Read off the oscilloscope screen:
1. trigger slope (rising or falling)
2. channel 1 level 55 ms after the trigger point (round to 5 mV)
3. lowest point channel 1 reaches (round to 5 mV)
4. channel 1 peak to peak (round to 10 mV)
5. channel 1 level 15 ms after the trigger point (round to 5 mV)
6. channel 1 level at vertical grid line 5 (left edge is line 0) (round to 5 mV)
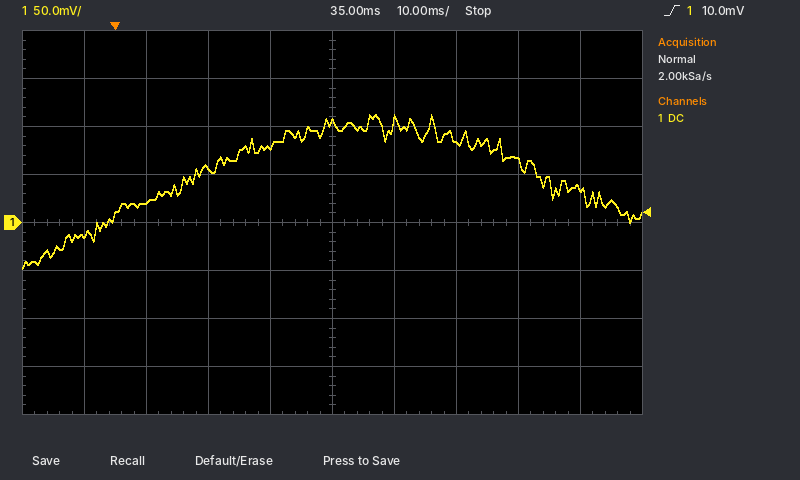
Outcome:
rising
85 mV
-50 mV
160 mV
55 mV
105 mV
